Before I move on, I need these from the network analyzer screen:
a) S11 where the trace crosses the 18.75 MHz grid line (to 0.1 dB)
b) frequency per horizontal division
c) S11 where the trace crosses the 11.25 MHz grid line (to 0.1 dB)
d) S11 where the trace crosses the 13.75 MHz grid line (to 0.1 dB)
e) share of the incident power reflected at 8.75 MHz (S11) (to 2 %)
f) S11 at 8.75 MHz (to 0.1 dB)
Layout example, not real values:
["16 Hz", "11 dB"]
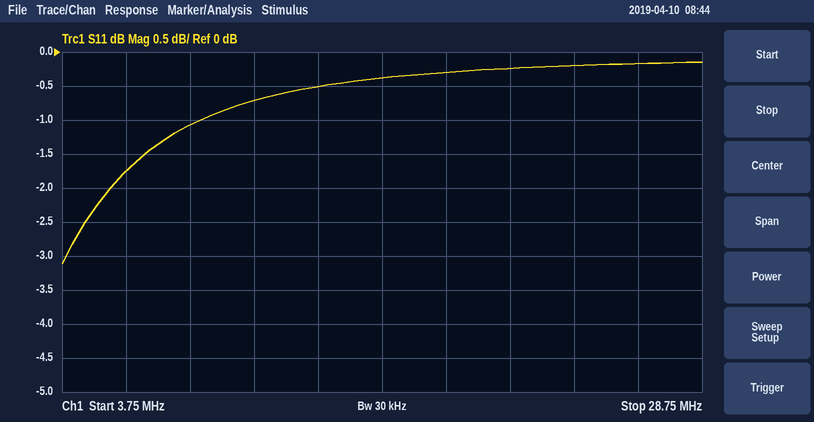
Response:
["-0.3 dB", "2.5 MHz", "-0.7 dB", "-0.5 dB", "78 %", "-1.1 dB"]
